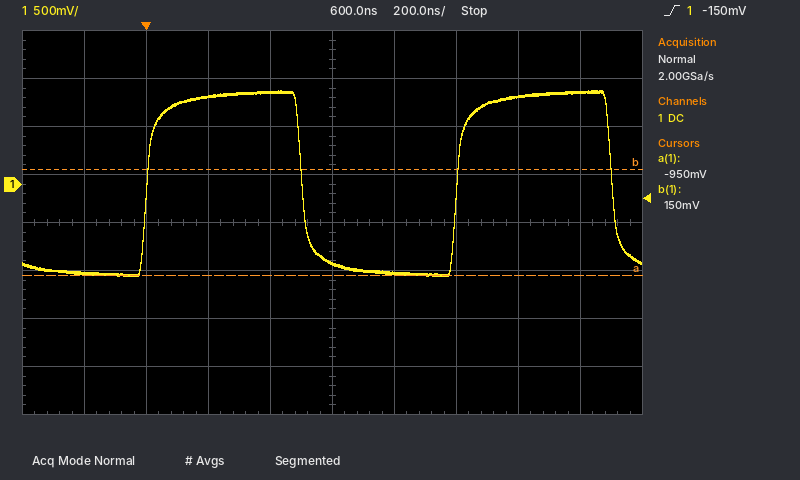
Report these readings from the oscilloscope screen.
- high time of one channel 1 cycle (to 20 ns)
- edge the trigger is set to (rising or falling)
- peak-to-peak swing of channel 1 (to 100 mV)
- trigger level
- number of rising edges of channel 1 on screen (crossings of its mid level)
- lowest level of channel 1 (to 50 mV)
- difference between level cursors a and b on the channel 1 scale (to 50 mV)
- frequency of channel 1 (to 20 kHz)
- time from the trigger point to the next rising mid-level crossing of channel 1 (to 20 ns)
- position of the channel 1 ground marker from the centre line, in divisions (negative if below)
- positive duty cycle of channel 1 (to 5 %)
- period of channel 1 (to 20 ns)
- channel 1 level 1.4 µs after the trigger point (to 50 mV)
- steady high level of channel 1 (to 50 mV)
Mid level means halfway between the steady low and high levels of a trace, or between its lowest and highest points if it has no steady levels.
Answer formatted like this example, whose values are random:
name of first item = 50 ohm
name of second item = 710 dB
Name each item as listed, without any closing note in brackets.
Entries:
high time of one channel 1 cycle = 500 ns
edge the trigger is set to = rising
peak-to-peak swing of channel 1 = 1.90 V
trigger level = -150 mV
number of rising edges of channel 1 on screen = 2
lowest level of channel 1 = -950 mV
difference between level cursors a and b on the channel 1 scale = 1.10 V
frequency of channel 1 = 1.00 MHz
time from the trigger point to the next rising mid-level crossing of channel 1 = 1.00 µs
position of the channel 1 ground marker from the centre line, in divisions = +0.8 div
positive duty cycle of channel 1 = 50 %
period of channel 1 = 1.00 µs
channel 1 level 1.4 µs after the trigger point = 950 mV
steady high level of channel 1 = 950 mV
